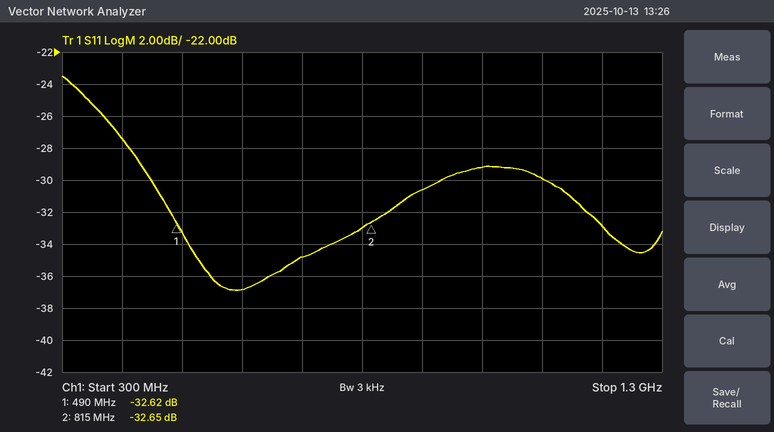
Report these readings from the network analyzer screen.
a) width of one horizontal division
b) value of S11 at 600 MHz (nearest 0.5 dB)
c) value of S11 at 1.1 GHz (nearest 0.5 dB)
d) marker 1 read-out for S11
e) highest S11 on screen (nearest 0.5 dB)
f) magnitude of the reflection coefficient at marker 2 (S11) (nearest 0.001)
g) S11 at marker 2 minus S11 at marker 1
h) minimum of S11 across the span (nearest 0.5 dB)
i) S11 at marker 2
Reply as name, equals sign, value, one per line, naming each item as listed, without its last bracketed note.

width of one horizontal division = 100 MHz
value of S11 at 600 MHz = -37.0 dB
value of S11 at 1.1 GHz = -30.0 dB
marker 1 read-out for S11 = -32.62 dB
highest S11 on screen = -23.5 dB
magnitude of the reflection coefficient at marker 2 (S11) = 0.023
S11 at marker 2 minus S11 at marker 1 = -0.03 dB
minimum of S11 across the span = -37.0 dB
S11 at marker 2 = -32.65 dB
